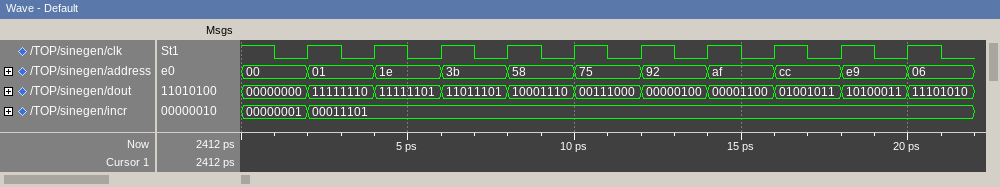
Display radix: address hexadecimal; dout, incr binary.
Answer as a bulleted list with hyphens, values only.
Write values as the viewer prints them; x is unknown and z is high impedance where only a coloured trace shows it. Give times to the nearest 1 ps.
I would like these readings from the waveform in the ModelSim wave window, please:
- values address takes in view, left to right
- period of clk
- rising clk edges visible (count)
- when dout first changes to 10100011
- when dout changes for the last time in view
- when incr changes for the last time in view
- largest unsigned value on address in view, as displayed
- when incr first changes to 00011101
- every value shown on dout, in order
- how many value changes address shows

- 00, 01, 1e, 3b, 58, 75, 92, af, cc, e9, 06
- 2 ps
- 10
- 18 ps
- 20 ps
- 2 ps
- e9
- 2 ps
- 00000000, 11111110, 11111101, 11011101, 10001110, 00111000, 00000100, 00001100, 01001011, 10100011, 11101010
- 10
